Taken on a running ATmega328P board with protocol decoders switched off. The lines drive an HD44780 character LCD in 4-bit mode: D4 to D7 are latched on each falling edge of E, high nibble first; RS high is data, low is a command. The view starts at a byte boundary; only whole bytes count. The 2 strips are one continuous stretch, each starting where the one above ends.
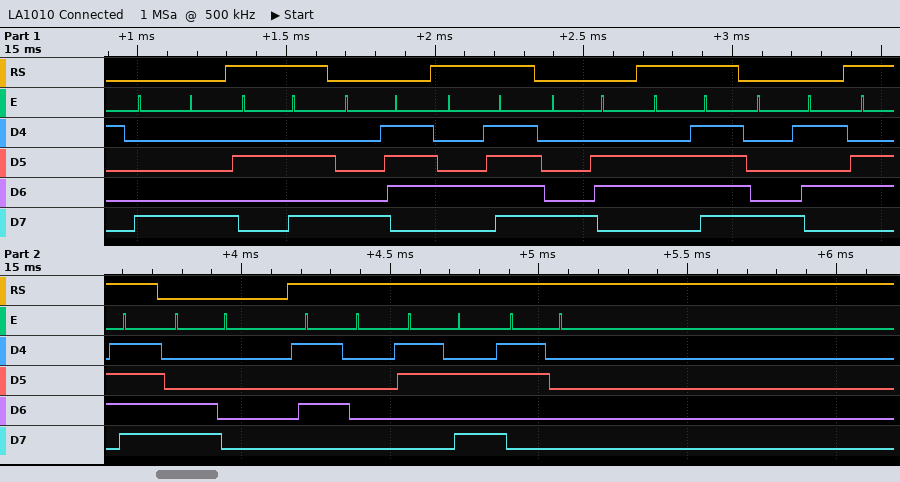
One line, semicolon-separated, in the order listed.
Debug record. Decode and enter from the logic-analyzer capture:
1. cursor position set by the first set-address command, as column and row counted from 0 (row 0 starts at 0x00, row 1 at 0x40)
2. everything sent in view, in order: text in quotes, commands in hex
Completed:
column 8, row 0; 0x88 "*" 0x87 "O" 0x86 "o" 0x85 "o" 0xC0 "P:0"
